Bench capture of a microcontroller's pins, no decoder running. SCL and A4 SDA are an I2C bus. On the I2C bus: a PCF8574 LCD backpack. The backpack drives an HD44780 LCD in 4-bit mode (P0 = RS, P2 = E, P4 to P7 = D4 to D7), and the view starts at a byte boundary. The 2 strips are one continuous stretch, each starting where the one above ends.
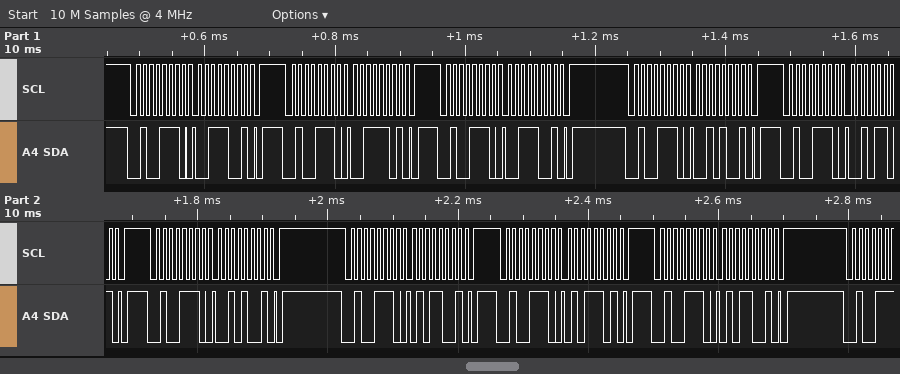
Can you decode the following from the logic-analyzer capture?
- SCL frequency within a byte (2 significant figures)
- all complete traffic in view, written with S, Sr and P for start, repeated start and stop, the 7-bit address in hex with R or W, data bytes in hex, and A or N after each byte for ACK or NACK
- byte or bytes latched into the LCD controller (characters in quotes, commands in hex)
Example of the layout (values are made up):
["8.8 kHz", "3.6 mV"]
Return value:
["100 kHz", "S 27W A 39 A P S 27W A 3D A P S 27W A 39 A P S 27W A 29 A P S 27W A 2D A P S 27W A 29 A P S 27W A 59 A P S 27W A 5D A P S 27W A 59 A P", "'2'"]
